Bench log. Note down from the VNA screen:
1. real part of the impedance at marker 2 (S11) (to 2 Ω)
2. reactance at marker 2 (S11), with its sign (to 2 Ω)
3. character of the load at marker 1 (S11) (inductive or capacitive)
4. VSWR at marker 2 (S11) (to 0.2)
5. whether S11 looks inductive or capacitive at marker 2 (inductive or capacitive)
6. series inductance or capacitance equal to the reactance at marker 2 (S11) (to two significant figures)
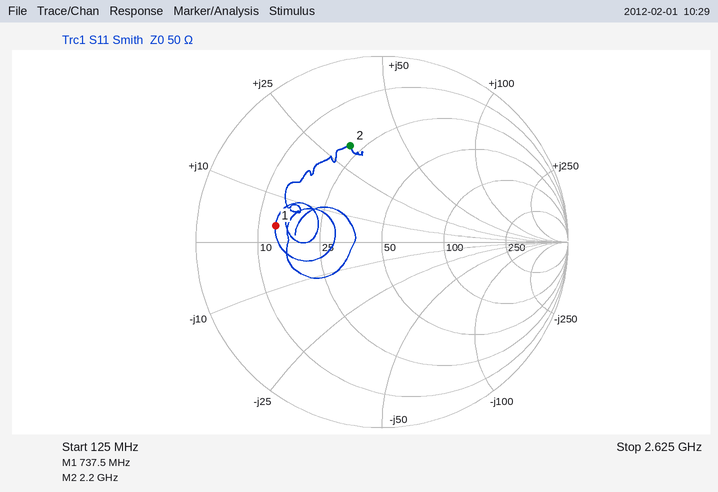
22 Ω
+32 Ω
inductive
3.4
inductive
2.3 nH
